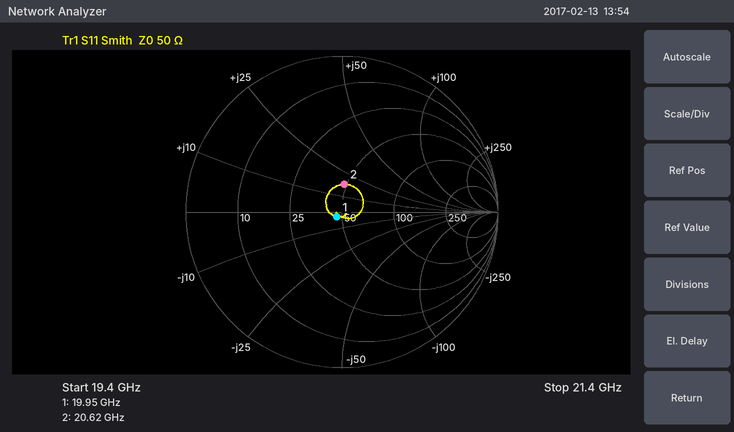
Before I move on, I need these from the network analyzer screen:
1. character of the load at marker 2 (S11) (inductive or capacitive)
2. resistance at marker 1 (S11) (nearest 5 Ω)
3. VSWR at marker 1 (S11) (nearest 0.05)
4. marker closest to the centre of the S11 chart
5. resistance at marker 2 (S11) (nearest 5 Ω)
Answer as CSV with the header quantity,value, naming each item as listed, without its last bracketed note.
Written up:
quantity,value
character of the load at marker 2 (S11),inductive
resistance at marker 1 (S11),45 Ω
VSWR at marker 1 (S11),1.10
marker closest to the centre of the S11 chart,marker 1
resistance at marker 2 (S11),50 Ω
